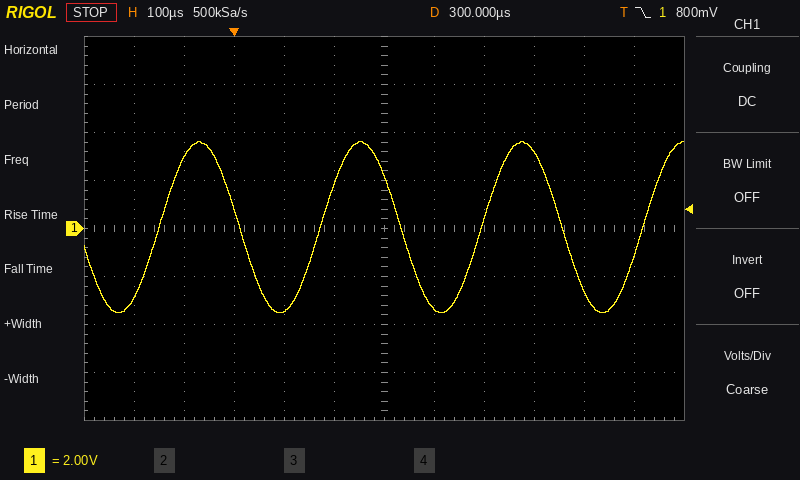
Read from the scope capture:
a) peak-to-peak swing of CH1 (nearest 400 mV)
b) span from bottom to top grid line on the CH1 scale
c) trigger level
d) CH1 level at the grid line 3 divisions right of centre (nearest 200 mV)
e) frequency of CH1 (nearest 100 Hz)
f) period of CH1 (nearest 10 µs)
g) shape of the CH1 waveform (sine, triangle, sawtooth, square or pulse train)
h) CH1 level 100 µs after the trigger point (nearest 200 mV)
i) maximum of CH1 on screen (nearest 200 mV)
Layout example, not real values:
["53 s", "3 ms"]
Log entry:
["7.2 V", "16 V", "800 mV", "3.2 V", "3.1 kHz", "320 µs", "sine", "-3.4 V", "3.6 V"]
